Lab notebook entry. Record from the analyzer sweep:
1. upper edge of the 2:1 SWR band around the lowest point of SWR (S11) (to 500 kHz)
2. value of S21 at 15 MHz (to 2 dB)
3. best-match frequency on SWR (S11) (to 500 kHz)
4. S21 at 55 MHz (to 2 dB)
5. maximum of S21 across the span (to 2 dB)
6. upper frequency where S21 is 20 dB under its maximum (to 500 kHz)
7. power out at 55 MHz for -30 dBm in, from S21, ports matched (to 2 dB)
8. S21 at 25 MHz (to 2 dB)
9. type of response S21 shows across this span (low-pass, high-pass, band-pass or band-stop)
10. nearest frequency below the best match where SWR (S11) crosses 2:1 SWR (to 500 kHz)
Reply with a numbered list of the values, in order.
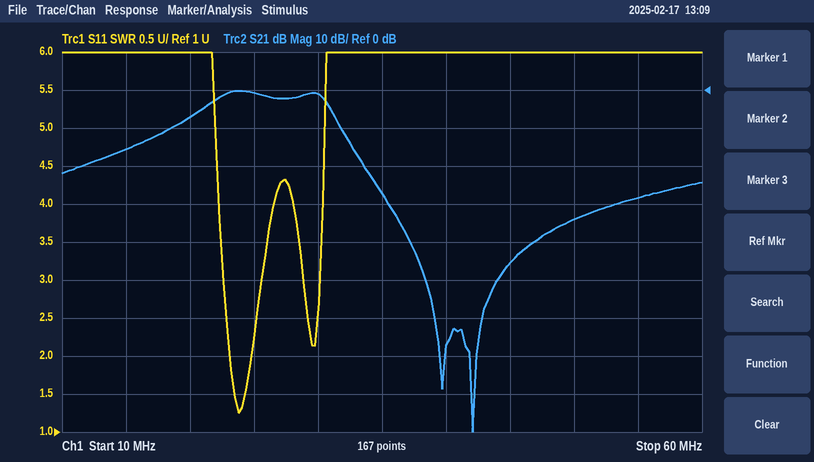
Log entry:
1. 25.0 MHz
2. -16 dB
3. 24.0 MHz
4. -28 dB
5. 0 dB
6. 33.5 MHz
7. -58 dBm
8. 0 dB
9. band-pass
10. 23.0 MHz
